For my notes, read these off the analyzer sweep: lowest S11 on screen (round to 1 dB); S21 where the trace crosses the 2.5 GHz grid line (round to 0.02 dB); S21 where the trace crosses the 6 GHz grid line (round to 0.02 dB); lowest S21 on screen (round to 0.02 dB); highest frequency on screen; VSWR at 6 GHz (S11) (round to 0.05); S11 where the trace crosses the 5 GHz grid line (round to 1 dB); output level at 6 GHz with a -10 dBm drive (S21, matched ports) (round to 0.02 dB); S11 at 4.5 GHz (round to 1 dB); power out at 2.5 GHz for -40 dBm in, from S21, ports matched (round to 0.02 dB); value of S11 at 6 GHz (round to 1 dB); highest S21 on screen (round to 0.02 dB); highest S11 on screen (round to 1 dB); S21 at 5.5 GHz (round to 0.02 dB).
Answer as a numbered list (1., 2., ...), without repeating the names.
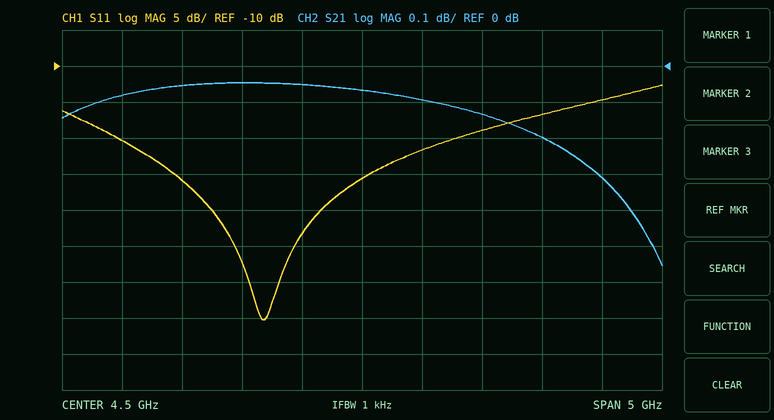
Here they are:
1. -45 dB
2. -0.08 dB
3. -0.20 dB
4. -0.56 dB
5. 7 GHz
6. 1.35
7. -22 dB
8. -10.20 dBm
9. -26 dB
10. -40.08 dBm
11. -17 dB
12. -0.04 dB
13. -13 dB
14. -0.14 dB
